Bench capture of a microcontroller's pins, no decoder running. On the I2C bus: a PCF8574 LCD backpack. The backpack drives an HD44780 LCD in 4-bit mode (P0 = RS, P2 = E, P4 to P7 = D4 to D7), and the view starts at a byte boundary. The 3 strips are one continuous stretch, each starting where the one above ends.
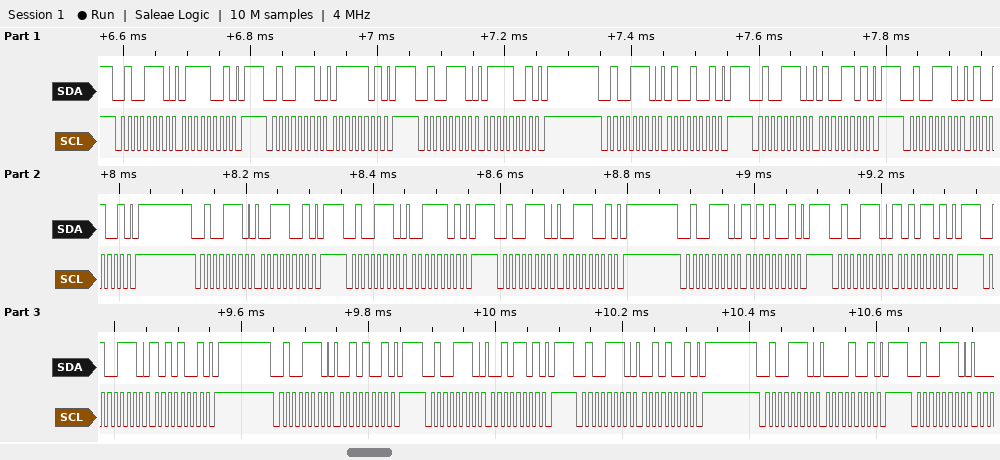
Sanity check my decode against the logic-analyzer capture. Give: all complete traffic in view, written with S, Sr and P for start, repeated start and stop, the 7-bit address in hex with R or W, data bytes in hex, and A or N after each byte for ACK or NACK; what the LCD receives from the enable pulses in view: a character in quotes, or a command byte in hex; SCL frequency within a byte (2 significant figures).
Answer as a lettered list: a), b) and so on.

a) S 27W A 79 A P S 27W A 7D A P S 27W A 79 A P S 27W A 49 A P S 27W A 4D A P S 27W A 49 A P S 27W A 39 A P S 27W A 3D A P S 27W A 39 A P S 27W A A9 A P S 27W A AD A P S 27W A A9 A P S 27W A 29 A P S 27W A 2D A P S 27W A 29 A P S 27W A 09 A P S 27W A
b) 't' ':'
c) 100 kHz
